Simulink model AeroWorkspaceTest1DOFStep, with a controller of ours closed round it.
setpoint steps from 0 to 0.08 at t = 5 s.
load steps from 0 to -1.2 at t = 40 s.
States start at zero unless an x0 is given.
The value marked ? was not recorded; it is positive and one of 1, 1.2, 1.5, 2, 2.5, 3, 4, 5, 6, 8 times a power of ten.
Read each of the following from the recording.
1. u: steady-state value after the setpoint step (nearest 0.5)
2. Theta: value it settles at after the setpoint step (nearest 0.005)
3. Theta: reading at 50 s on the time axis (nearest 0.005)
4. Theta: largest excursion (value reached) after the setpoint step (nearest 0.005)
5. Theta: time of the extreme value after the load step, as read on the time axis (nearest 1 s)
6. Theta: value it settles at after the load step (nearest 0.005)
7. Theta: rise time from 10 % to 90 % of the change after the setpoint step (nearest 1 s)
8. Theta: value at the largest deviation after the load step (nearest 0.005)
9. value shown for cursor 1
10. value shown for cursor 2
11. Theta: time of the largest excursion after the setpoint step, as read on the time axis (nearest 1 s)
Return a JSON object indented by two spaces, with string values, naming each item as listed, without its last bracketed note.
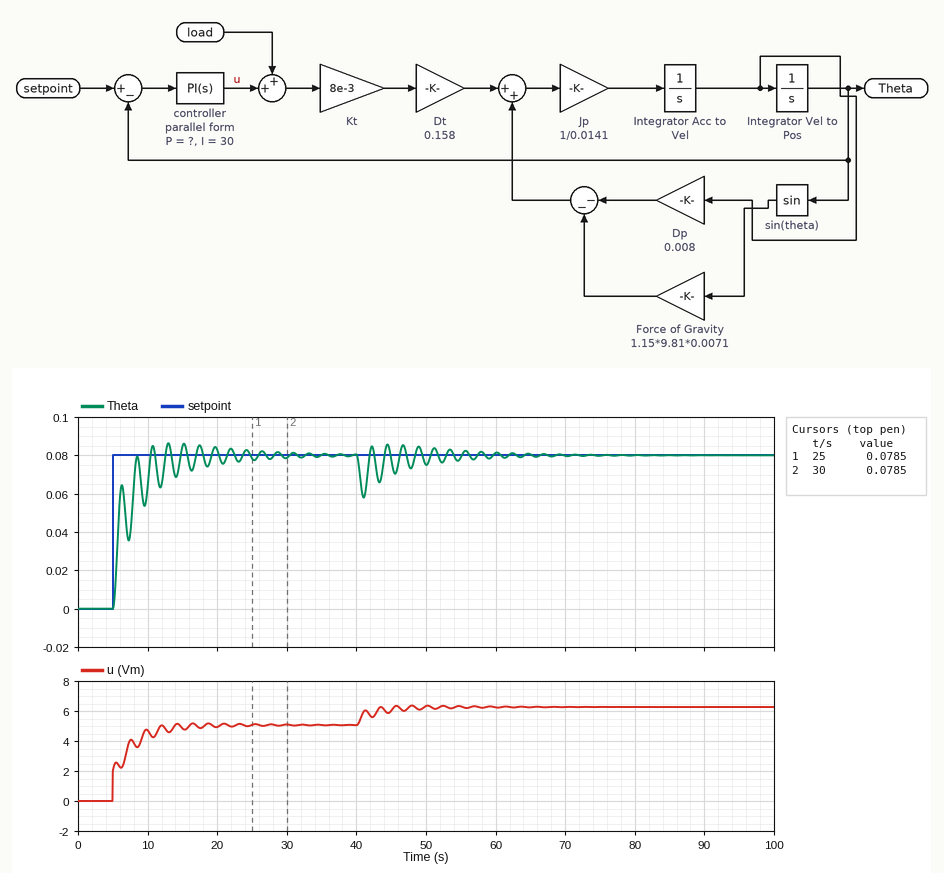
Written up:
{
  "u: steady-state value after the setpoint step": "5.0",
  "Theta: value it settles at after the setpoint step": "0.080",
  "Theta: reading at 50 s on the time axis": "0.075",
  "Theta: largest excursion (value reached) after the setpoint step": "0.085",
  "Theta: time of the extreme value after the load step, as read on the time axis": "41 s",
  "Theta: value it settles at after the load step": "0.080",
  "Theta: rise time from 10 % to 90 % of the change after the setpoint step": "3 s",
  "Theta: value at the largest deviation after the load step": "0.060",
  "value shown for cursor 1": "0.0785",
  "value shown for cursor 2": "0.0785",
  "Theta: time of the largest excursion after the setpoint step, as read on the time axis": "13 s"
}
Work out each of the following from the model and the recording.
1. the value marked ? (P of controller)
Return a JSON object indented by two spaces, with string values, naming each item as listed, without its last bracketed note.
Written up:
{
  "the value marked ?": "25"
}
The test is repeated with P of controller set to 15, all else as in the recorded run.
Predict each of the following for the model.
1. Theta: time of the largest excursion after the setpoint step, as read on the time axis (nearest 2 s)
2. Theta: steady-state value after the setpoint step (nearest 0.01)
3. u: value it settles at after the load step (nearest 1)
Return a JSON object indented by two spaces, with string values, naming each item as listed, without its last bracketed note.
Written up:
{
  "Theta: time of the largest excursion after the setpoint step, as read on the time axis": "14 s",
  "Theta: steady-state value after the setpoint step": "0.08",
  "u: value it settles at after the load step": "6"
}
